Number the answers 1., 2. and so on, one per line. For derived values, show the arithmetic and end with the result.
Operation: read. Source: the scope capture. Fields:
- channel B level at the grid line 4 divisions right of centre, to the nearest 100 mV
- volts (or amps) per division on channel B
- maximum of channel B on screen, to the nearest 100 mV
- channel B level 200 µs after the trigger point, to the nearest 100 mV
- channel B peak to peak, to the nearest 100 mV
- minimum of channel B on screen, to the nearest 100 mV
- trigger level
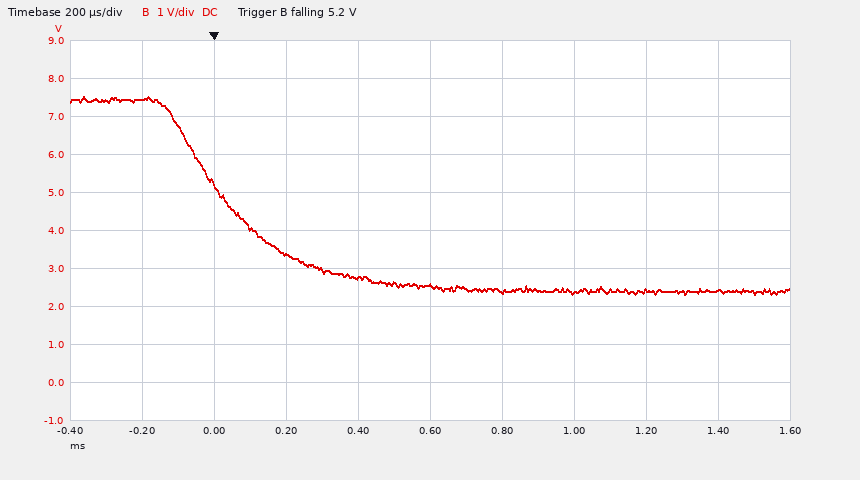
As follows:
1. 2.4 V
2. 1 V
3. 7.5 V
4. 3.4 V
5. 7.5 V − (2.3 V) = 5.2 V
6. 2.3 V
7. 5.2 V
